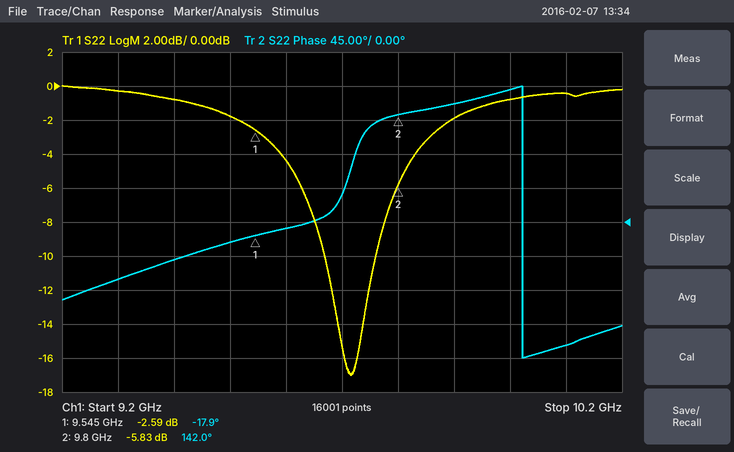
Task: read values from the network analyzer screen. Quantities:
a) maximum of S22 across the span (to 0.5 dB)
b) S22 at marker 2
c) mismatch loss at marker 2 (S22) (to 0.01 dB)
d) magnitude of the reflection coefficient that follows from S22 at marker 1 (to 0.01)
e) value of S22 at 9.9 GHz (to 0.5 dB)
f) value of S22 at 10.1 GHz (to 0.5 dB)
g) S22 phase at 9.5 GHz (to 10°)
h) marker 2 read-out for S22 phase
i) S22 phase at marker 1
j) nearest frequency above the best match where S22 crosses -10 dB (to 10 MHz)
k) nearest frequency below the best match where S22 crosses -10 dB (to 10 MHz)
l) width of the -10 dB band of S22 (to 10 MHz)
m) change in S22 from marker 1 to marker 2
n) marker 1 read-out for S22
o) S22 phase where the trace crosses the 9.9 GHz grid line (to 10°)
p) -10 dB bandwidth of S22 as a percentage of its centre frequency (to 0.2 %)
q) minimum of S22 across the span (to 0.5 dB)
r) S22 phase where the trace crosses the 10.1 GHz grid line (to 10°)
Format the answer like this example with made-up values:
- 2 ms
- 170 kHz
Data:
- 0.0 dB
- -5.83 dB
- 1.31 dB
- 0.74
- -2.0 dB
- -0.5 dB
- -30°
- 142.0°
- -17.9°
- 9.76 GHz
- 9.67 GHz
- 90 MHz
- -3.24 dB
- -2.59 dB
- 160°
- 1.0 %
- -17.0 dB
- -160°
